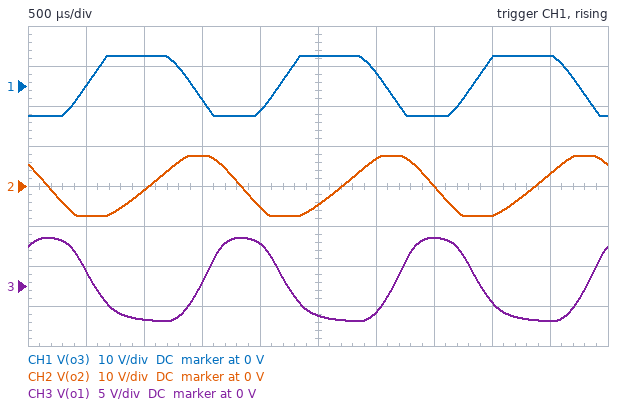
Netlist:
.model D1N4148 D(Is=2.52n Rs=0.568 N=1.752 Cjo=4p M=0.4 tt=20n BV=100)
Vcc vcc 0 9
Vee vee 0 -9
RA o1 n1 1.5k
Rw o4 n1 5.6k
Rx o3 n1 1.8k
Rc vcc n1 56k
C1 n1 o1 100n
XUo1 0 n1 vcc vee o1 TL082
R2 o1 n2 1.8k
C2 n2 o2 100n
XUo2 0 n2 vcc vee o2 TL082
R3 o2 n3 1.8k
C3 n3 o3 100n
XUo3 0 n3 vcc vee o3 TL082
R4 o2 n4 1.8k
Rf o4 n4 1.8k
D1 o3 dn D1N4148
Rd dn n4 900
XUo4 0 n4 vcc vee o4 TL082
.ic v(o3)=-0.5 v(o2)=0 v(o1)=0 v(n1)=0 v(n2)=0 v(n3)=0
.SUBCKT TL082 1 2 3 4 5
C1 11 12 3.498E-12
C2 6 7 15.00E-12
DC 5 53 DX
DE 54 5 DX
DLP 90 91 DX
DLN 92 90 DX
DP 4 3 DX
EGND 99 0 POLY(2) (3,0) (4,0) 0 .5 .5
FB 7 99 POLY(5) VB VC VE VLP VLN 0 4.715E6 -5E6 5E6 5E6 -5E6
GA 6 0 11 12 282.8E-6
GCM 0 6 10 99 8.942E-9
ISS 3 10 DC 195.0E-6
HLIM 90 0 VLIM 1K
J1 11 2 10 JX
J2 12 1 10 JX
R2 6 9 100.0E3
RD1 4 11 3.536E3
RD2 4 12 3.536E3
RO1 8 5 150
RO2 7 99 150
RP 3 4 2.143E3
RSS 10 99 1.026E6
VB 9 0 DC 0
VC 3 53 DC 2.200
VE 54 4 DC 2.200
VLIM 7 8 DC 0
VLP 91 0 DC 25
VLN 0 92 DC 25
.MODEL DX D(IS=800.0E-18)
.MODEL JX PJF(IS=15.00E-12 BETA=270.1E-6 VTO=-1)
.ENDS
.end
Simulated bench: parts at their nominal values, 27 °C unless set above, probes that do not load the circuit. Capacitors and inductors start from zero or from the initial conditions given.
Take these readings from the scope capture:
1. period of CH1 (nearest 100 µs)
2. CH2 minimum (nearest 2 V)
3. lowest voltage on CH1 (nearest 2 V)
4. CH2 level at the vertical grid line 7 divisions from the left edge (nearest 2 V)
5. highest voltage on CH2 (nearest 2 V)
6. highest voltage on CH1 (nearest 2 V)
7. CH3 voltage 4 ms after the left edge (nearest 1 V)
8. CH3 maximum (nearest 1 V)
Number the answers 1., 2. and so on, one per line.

1. 1.7 ms
2. -8 V
3. -8 V
4. 0 V
5. 8 V
6. 8 V
7. -2 V
8. 6 V
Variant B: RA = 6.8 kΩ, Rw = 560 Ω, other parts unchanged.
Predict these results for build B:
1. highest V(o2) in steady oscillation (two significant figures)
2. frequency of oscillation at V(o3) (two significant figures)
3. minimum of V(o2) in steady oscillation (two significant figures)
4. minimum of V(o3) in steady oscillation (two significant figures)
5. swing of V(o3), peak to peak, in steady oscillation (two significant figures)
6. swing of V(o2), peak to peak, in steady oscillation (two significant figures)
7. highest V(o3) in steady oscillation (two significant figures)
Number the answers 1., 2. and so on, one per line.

1. 1.4 V
2. 1.6 kHz
3. -1.4 V
4. -990 mV
5. 1.5 V
6. 2.8 V
7. 550 mV
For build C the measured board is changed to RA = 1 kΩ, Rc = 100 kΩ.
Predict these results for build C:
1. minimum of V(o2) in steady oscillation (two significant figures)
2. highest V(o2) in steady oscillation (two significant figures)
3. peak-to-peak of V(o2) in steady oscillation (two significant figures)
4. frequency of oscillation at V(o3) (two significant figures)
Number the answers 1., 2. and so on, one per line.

1. -6.4 V
2. 5.7 V
3. 12 V
4. 550 Hz
